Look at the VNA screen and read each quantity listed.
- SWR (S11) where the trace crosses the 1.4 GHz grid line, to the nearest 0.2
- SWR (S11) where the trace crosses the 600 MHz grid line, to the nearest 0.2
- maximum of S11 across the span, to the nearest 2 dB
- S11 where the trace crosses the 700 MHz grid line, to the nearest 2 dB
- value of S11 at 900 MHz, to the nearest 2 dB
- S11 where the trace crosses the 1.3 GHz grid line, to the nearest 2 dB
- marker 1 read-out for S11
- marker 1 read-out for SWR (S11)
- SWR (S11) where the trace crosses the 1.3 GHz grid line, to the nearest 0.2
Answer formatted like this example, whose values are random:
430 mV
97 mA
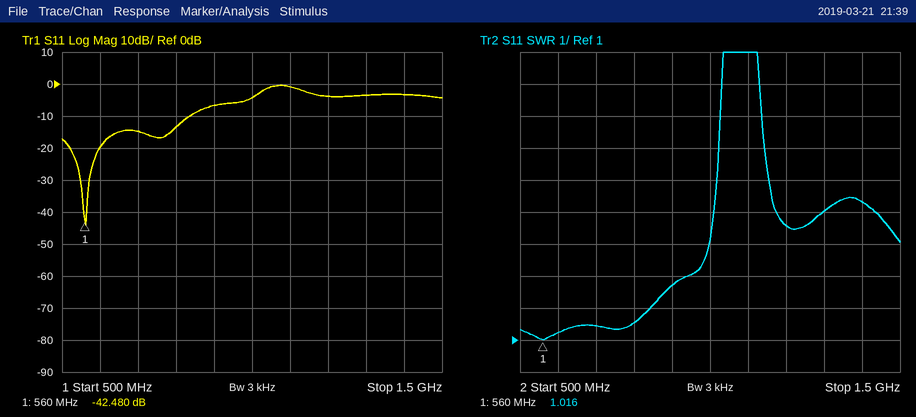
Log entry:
5.4
1.2
0 dB
-14 dB
-6 dB
-4 dB
-42.480 dB
1.016
5.0
